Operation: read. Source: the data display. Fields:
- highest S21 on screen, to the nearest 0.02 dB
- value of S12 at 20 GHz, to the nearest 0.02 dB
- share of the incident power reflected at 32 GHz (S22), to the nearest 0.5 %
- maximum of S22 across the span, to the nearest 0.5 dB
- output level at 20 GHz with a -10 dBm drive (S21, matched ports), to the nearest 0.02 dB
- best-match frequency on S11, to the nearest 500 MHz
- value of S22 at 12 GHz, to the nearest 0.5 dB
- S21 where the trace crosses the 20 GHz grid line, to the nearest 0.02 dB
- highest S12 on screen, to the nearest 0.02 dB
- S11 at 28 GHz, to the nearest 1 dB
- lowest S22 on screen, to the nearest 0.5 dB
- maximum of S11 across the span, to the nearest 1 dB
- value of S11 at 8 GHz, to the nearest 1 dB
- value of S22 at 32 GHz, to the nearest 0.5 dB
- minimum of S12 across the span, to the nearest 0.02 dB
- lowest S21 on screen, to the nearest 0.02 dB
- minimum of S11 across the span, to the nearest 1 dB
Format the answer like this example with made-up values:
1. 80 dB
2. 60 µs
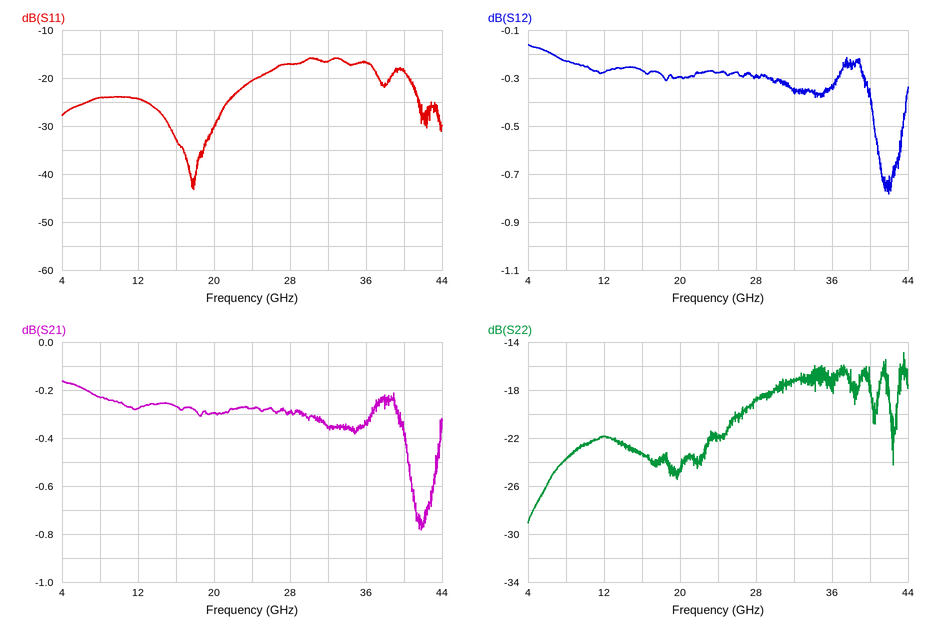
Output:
1. -0.16 dB
2. -0.30 dB
3. 2.0 %
4. -15.0 dB
5. -10.30 dBm
6. 18.0 GHz
7. -22.0 dB
8. -0.30 dB
9. -0.16 dB
10. -17 dB
11. -29.0 dB
12. -16 dB
13. -24 dB
14. -17.0 dB
15. -0.78 dB
16. -0.78 dB
17. -43 dB
